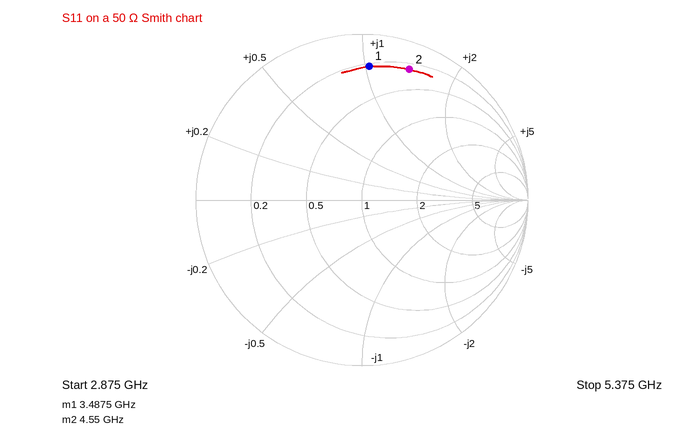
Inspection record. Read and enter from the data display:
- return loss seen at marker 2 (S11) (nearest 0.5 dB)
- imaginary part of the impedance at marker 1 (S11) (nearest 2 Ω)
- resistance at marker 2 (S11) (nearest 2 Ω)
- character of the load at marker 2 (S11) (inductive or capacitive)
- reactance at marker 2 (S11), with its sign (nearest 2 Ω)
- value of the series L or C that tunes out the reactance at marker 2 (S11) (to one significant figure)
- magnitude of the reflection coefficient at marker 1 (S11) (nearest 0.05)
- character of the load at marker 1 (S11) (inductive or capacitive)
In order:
1.5 dB
+52 Ω
14 Ω
inductive
+70 Ω
500 fF
0.80
inductive
